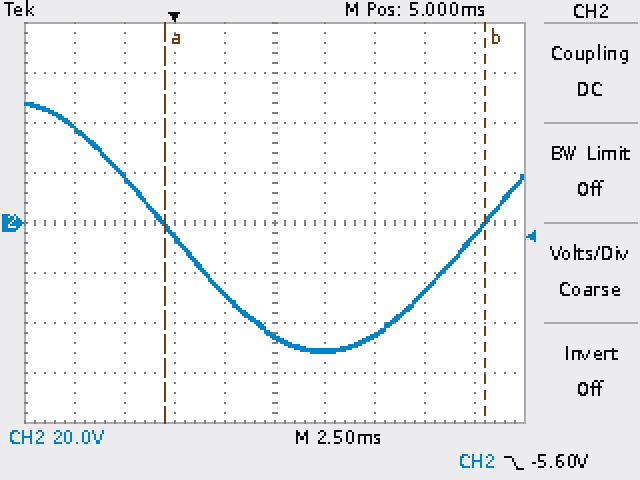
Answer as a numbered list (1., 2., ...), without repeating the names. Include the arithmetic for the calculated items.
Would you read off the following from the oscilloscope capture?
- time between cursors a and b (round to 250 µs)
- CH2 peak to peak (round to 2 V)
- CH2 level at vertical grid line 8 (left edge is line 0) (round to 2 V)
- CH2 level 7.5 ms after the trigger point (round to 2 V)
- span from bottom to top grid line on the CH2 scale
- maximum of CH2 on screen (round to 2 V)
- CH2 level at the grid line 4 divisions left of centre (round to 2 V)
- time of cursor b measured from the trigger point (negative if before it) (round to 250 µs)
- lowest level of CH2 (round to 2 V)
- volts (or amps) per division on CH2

1. 16.00 ms
2. 48 V − (-52 V) = 100 V
3. -28 V
4. -52 V
5. 160 V
6. 48 V
7. 38 V
8. +15.50 ms
9. -52 V
10. 20 V
